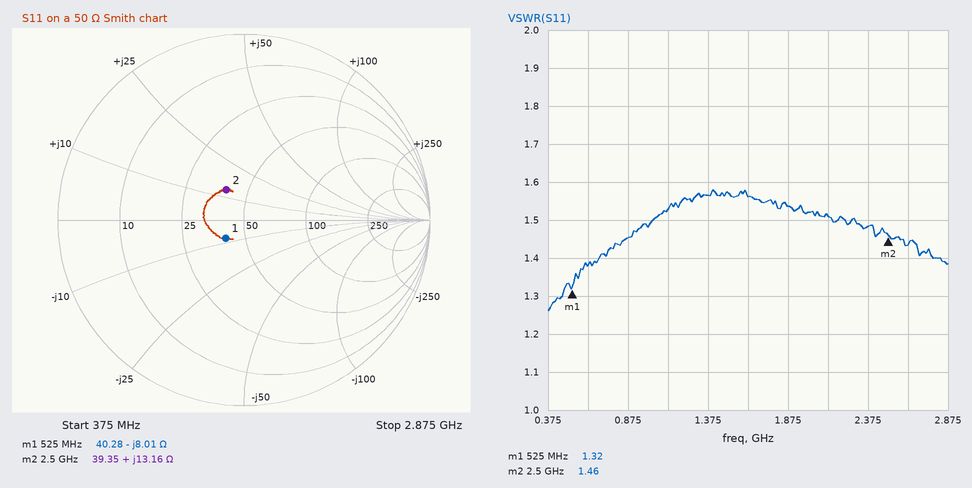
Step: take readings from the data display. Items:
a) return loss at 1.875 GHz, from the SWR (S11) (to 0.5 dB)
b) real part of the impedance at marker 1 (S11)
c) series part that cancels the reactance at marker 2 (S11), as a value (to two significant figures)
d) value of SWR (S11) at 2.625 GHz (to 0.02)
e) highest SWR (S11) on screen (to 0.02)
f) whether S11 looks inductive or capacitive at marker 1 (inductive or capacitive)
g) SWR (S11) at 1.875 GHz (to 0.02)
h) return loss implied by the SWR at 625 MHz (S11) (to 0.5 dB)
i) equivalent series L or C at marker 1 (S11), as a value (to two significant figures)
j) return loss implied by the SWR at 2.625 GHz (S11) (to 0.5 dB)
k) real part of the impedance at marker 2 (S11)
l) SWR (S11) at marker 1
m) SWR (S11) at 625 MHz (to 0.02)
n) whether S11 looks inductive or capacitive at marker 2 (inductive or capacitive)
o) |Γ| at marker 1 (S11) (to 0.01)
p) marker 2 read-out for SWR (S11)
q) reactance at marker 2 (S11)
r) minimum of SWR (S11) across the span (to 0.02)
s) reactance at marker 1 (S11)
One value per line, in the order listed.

13.5 dB
40.28 Ω
4.8 pF
1.44
1.58
capacitive
1.54
16.0 dB
38 pF
15.0 dB
39.35 Ω
1.32
1.38
inductive
0.14
1.46
+13.16 Ω
1.26
-8.01 Ω
